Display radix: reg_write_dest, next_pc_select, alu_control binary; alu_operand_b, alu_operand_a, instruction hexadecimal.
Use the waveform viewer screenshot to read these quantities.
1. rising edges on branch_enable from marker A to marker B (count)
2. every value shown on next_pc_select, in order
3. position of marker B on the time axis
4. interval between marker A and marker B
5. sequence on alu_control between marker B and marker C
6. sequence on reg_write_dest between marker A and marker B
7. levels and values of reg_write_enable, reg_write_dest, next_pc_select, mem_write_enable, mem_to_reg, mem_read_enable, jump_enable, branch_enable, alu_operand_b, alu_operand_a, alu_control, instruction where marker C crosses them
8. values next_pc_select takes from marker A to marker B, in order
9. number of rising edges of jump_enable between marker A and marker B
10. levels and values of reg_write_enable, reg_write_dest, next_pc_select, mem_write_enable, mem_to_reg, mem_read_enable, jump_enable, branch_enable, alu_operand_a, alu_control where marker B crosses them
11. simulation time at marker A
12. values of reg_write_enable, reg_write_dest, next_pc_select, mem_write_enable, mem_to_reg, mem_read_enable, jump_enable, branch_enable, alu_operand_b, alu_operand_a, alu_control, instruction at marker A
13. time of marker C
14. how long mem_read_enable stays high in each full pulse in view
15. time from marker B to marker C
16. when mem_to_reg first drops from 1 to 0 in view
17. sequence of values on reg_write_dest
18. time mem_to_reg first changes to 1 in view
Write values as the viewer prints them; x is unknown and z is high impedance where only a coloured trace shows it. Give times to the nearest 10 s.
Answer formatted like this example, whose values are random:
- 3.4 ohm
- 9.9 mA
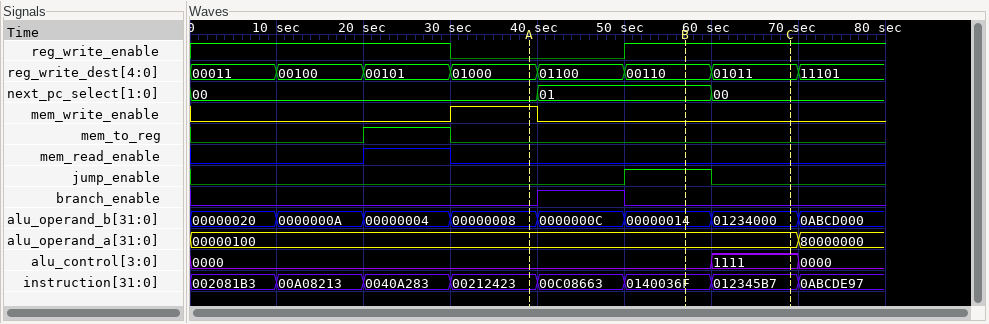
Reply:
- 1
- 00, 01, 00
- 60 s
- 20 s
- 0000, 1111
- 01000, 01100, 00110
- reg_write_enable=1, reg_write_dest=01011, next_pc_select=00, mem_write_enable=0, mem_to_reg=0, mem_read_enable=0, jump_enable=0, branch_enable=0, alu_operand_b=01234000, alu_operand_a=00000100, alu_control=1111, instruction=012345B7
- 00, 01
- 1
- reg_write_enable=1, reg_write_dest=00110, next_pc_select=01, mem_write_enable=0, mem_to_reg=0, mem_read_enable=0, jump_enable=1, branch_enable=0, alu_operand_a=00000100, alu_control=0000
- 40 s
- reg_write_enable=0, reg_write_dest=01000, next_pc_select=00, mem_write_enable=1, mem_to_reg=0, mem_read_enable=0, jump_enable=0, branch_enable=0, alu_operand_b=00000008, alu_operand_a=00000100, alu_control=0000, instruction=00212423
- 70 s
- 10 s
- 10 s
- 30 s
- 00011, 00100, 00101, 01000, 01100, 00110, 01011, 11101
- 20 s
